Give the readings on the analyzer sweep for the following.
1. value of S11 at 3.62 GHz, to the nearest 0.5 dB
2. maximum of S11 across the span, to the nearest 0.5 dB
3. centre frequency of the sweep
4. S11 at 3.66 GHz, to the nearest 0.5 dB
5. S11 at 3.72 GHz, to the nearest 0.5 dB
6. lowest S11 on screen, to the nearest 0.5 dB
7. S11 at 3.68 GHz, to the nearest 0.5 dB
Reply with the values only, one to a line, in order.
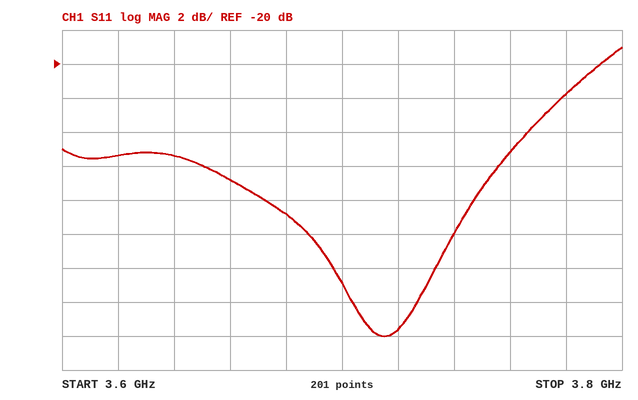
-25.5 dB
-19.0 dB
3.7 GHz
-27.0 dB
-35.5 dB
-36.0 dB
-29.0 dB
